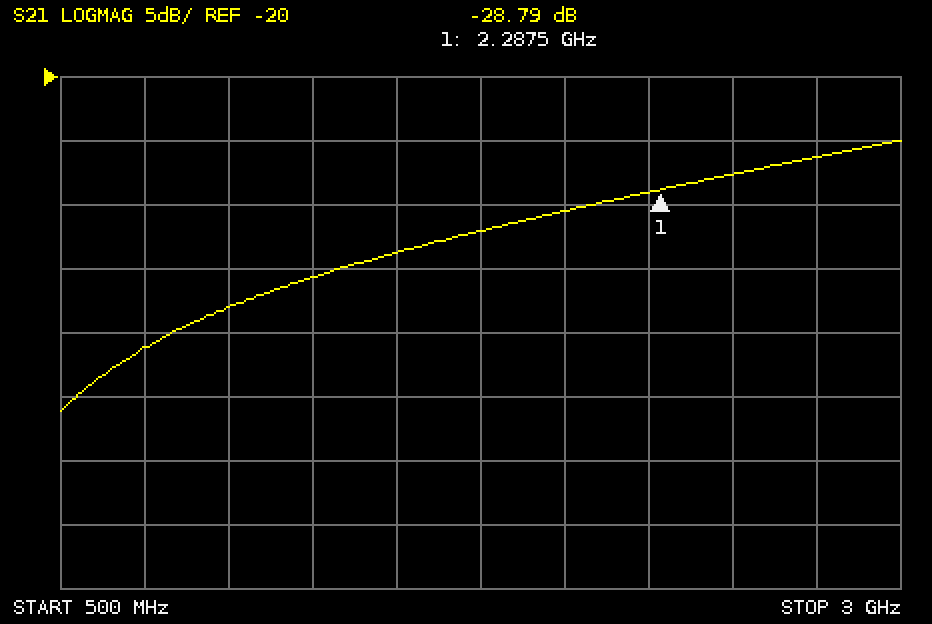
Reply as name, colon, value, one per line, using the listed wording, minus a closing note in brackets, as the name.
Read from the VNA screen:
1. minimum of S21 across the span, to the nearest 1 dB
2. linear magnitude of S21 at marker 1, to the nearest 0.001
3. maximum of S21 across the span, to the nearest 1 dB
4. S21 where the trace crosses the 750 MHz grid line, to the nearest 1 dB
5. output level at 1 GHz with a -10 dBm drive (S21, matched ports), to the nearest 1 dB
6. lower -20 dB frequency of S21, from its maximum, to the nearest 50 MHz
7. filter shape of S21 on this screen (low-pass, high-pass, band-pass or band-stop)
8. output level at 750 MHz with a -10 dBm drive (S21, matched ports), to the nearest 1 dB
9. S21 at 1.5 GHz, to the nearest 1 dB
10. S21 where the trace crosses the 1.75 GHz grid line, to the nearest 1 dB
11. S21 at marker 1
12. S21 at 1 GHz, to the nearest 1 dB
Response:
minimum of S21 across the span, to the nearest 1 dB: -46 dB
linear magnitude of S21 at marker 1, to the nearest 0.001: 0.036
maximum of S21 across the span, to the nearest 1 dB: -25 dB
S21 where the trace crosses the 750 MHz grid line, to the nearest 1 dB: -41 dB
output level at 1 GHz with a -10 dBm drive (S21, matched ports), to the nearest 1 dB: -48 dBm
lower -20 dB frequency of S21, from its maximum, to the nearest 50 MHz: 550 MHz
filter shape of S21 on this screen: high-pass
output level at 750 MHz with a -10 dBm drive (S21, matched ports), to the nearest 1 dB: -51 dBm
S21 at 1.5 GHz, to the nearest 1 dB: -34 dB
S21 where the trace crosses the 1.75 GHz grid line, to the nearest 1 dB: -32 dB
S21 at marker 1: -28.79 dB
S21 at 1 GHz, to the nearest 1 dB: -38 dB
